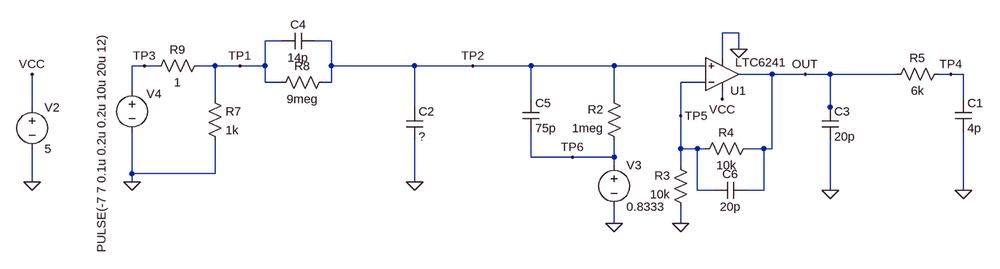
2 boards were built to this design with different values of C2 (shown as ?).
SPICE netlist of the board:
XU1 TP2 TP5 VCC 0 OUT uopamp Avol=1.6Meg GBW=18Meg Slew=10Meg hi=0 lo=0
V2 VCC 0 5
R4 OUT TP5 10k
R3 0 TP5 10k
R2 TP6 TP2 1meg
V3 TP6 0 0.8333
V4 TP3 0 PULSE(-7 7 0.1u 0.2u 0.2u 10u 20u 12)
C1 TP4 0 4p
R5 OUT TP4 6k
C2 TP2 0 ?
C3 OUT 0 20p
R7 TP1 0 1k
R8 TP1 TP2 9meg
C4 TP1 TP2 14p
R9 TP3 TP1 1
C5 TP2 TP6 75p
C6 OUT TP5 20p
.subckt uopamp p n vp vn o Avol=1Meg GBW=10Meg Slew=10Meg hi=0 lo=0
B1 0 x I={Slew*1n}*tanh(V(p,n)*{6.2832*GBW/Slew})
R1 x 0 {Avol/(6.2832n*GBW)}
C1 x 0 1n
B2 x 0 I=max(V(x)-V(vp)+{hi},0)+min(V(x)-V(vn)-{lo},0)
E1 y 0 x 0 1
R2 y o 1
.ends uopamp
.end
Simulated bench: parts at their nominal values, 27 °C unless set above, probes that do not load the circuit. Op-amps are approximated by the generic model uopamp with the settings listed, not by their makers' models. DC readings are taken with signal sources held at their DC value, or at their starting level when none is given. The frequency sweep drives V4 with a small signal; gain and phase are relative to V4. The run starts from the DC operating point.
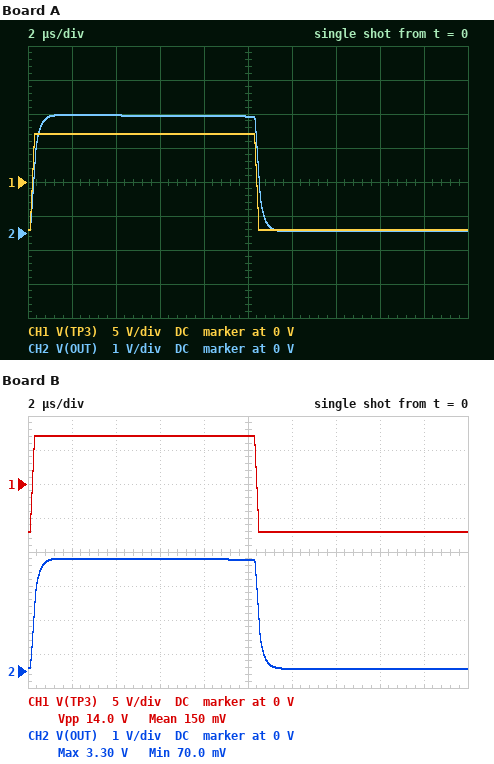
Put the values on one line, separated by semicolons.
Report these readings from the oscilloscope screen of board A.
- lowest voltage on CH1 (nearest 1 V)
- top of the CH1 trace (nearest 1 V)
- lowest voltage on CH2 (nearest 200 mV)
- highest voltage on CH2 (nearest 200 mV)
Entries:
-7 V; 7 V; 0 V; 3.4 V
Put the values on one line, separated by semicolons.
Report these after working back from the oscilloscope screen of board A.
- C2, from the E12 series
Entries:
27 pF
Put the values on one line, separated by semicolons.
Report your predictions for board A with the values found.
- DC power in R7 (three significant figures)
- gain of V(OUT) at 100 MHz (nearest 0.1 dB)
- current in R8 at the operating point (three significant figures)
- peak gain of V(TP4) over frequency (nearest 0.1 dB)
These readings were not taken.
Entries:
48.9 mW; -33.4 dB; 783 nA; -12.4 dB
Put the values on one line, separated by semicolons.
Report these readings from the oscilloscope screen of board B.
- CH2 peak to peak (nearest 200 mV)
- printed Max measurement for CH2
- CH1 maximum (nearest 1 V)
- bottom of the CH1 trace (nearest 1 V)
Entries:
3.2 V; 3.30 V; 7 V; -7 V
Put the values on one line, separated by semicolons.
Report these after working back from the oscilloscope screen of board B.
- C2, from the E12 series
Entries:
33 pF
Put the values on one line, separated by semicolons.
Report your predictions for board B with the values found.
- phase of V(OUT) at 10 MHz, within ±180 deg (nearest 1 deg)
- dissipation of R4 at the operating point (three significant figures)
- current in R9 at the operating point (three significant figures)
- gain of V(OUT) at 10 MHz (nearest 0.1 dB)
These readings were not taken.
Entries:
-33 deg; 257 nW; 6.99 mA; -20.2 dB
